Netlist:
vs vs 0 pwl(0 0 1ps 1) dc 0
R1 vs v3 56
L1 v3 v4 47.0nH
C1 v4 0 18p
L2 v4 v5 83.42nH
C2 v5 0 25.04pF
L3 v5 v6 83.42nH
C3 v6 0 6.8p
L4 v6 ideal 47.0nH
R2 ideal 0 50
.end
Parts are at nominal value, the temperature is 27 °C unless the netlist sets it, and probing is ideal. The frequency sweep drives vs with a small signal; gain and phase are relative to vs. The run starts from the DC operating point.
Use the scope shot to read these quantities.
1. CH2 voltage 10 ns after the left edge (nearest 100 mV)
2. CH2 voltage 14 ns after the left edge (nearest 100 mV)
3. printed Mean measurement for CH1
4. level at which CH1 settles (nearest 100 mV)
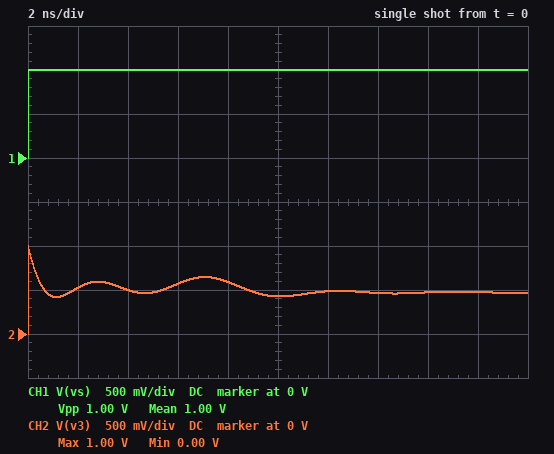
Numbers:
400 mV
500 mV
1.00 V
1.0 V
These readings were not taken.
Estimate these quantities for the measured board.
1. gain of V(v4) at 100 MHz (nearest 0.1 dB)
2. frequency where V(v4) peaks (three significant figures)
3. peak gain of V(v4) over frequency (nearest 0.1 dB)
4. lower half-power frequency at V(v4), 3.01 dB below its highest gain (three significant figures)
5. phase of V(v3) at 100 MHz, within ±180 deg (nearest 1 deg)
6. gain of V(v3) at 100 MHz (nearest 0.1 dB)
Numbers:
-5.4 dB
209 MHz
2.5 dB
180 MHz
-6 deg
-8.7 dB
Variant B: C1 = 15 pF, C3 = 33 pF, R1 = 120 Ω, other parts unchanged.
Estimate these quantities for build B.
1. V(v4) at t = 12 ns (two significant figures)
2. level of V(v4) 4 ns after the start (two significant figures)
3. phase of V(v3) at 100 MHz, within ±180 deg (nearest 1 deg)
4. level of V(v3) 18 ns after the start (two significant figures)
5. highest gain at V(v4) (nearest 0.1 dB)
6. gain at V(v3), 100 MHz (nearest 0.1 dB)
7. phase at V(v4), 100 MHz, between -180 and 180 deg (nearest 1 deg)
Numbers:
300 mV
250 mV
15 deg
280 mV
0.3 dB
-7.4 dB
-5 deg
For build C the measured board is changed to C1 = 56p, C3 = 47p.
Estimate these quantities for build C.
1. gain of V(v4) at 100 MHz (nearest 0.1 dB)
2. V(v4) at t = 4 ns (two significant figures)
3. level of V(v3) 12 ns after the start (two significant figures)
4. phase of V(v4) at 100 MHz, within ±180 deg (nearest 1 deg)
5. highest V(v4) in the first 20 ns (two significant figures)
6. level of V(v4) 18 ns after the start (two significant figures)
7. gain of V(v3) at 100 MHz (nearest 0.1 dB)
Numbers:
-4.6 dB
510 mV
440 mV
-65 deg
520 mV
480 mV
-13.2 dB
